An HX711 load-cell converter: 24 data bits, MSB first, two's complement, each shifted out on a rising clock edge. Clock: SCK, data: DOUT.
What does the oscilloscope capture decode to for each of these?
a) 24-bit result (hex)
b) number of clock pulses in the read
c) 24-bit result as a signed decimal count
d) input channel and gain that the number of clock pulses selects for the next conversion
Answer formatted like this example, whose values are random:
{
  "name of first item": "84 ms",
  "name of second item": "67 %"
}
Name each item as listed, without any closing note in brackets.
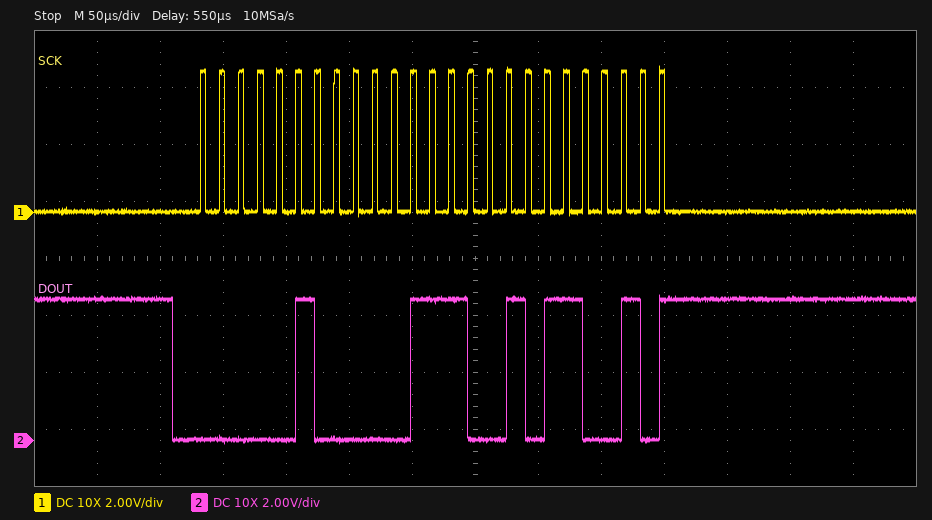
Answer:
{
  "24-bit result": "0x041CB2",
  "number of clock pulses in the read": "25",
  "24-bit result as a signed decimal count": "269490",
  "input channel and gain that the number of clock pulses selects for the next conversion": "channel A, gain 128"
}
